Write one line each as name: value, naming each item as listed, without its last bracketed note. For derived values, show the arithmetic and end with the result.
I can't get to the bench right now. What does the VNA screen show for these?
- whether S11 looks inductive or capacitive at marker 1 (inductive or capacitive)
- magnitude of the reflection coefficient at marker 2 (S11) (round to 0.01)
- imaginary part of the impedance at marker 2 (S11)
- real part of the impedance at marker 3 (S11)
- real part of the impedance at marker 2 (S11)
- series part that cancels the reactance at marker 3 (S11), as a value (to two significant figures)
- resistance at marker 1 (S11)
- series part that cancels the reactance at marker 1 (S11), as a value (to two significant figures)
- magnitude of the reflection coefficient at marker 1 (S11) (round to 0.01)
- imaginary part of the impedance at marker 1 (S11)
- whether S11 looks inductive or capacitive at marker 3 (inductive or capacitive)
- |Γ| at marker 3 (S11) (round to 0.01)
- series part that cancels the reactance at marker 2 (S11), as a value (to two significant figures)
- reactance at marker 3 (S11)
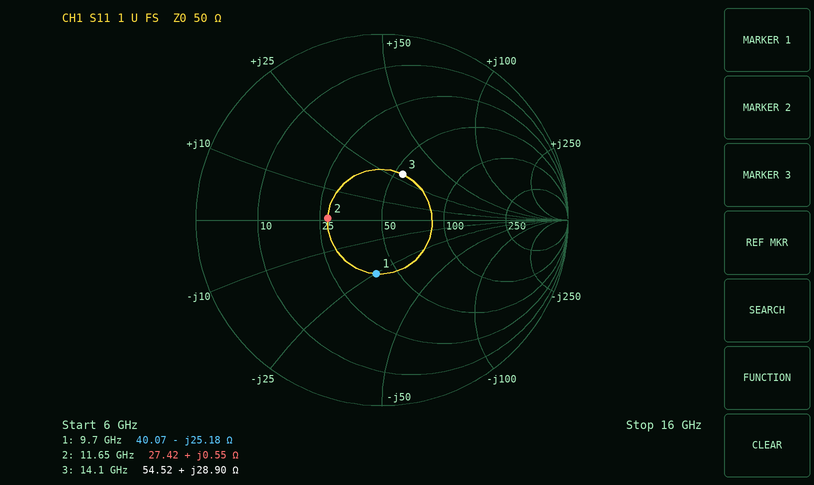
whether S11 looks inductive or capacitive at marker 1: capacitive
magnitude of the reflection coefficient at marker 2 (S11): 0.29
imaginary part of the impedance at marker 2: +0.55 Ω
real part of the impedance at marker 3: 54.52 Ω
real part of the impedance at marker 2: 27.42 Ω
series part that cancels the reactance at marker 3 (S11), as a value: C = 1/(2π × 14.1 GHz × 28.9 Ω) ≈ 391 fF, so 390 fF to two significant figures
resistance at marker 1: 40.07 Ω
series part that cancels the reactance at marker 1 (S11), as a value: L = 25.18 Ω/(2π × 9.7 GHz) ≈ 413 pH, so 410 pH to two significant figures
magnitude of the reflection coefficient at marker 1 (S11): 0.29
imaginary part of the impedance at marker 1: -25.18 Ω
whether S11 looks inductive or capacitive at marker 3: inductive
|Γ| at marker 3 (S11): 0.27
series part that cancels the reactance at marker 2 (S11), as a value: C = 1/(2π × 11.65 GHz × 0.55 Ω) ≈ 25 pF
reactance at marker 3: +28.90 Ω
